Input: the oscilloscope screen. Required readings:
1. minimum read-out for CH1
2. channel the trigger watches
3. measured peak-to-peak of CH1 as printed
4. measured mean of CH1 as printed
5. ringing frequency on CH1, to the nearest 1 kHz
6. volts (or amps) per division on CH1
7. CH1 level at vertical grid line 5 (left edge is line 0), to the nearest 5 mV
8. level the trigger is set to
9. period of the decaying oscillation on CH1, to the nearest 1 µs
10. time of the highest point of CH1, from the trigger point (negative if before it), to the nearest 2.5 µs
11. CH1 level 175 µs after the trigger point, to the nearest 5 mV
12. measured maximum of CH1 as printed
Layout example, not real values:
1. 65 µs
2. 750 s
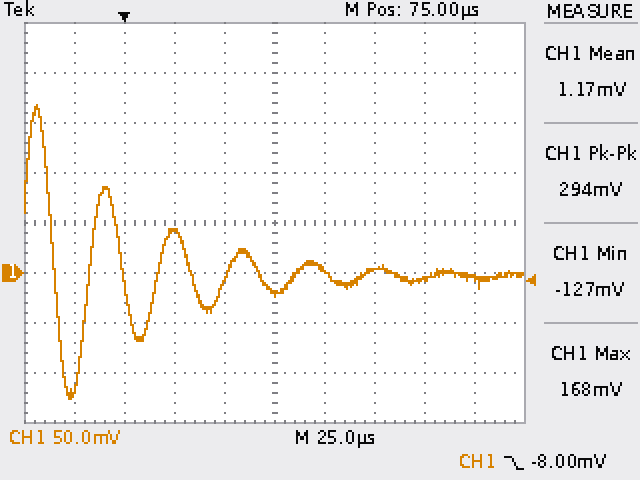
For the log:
1. -127 mV
2. CH1
3. 294 mV
4. 1.17 mV
5. 29 kHz
6. 50 mV
7. -20 mV
8. -8.00 mV
9. 34 µs
10. -42.5 µs
11. -5 mV
12. 168 mV
